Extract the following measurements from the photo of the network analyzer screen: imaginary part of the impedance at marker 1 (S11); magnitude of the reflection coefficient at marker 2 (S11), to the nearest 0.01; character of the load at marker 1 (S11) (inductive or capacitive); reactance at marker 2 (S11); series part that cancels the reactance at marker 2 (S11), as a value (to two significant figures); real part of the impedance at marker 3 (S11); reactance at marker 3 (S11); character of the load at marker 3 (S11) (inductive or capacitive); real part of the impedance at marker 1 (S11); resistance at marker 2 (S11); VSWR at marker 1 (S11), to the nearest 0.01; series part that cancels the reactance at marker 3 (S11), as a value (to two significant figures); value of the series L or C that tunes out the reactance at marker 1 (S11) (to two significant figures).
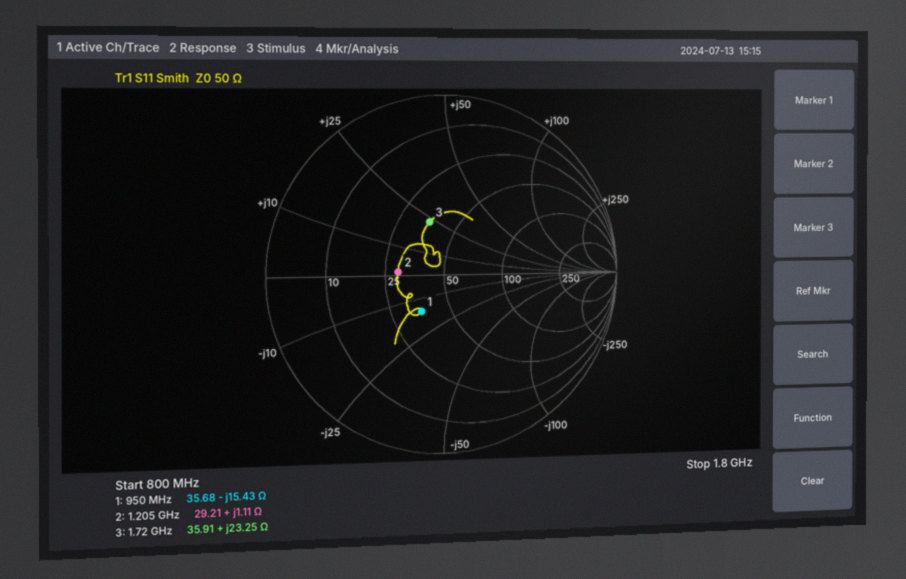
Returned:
-15.43 Ω
0.26
capacitive
+1.11 Ω
120 pF
35.91 Ω
+23.25 Ω
inductive
35.68 Ω
29.21 Ω
1.64
4.0 pF
2.6 nH
